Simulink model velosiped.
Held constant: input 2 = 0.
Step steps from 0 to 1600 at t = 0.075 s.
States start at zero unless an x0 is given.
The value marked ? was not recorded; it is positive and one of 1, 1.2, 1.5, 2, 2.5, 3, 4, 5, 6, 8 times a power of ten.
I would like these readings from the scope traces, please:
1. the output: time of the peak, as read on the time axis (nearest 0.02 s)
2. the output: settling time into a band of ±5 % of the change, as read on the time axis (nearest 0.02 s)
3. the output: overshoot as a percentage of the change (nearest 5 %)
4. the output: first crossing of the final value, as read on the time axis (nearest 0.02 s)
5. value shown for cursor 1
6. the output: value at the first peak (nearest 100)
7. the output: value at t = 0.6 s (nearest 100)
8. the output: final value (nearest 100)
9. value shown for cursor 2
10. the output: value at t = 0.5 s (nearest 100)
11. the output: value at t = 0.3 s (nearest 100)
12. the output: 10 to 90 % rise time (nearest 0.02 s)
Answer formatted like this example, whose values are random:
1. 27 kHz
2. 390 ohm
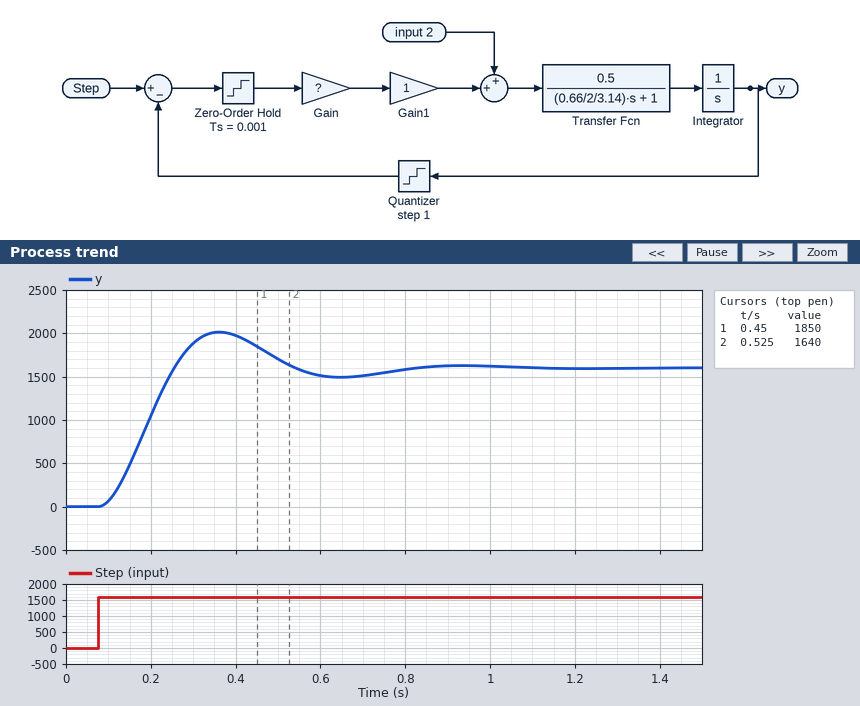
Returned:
1. 0.36 s
2. 0.72 s
3. 25 %
4. 0.26 s
5. 1850
6. 2000
7. 1500
8. 1600
9. 1640
10. 1700
11. 1900
12. 0.12 s
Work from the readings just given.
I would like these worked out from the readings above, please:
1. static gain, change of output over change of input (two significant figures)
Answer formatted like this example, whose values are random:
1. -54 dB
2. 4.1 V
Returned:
1. 1.0
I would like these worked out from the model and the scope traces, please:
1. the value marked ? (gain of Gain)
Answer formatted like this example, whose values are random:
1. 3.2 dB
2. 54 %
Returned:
1. 30
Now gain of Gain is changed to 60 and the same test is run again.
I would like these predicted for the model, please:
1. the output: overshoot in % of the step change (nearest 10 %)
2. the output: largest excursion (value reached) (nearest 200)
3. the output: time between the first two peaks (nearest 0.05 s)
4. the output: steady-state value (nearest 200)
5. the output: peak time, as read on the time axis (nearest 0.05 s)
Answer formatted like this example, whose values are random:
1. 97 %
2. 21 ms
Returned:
1. 40 %
2. 2200
3. 0.40 s
4. 1600
5. 0.25 s
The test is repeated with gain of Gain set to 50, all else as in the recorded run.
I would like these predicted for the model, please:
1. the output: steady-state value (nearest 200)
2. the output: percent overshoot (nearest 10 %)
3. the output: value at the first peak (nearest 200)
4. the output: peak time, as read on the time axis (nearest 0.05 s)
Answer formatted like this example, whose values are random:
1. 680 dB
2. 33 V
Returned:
1. 1600
2. 40 %
3. 2200
4. 0.30 s
